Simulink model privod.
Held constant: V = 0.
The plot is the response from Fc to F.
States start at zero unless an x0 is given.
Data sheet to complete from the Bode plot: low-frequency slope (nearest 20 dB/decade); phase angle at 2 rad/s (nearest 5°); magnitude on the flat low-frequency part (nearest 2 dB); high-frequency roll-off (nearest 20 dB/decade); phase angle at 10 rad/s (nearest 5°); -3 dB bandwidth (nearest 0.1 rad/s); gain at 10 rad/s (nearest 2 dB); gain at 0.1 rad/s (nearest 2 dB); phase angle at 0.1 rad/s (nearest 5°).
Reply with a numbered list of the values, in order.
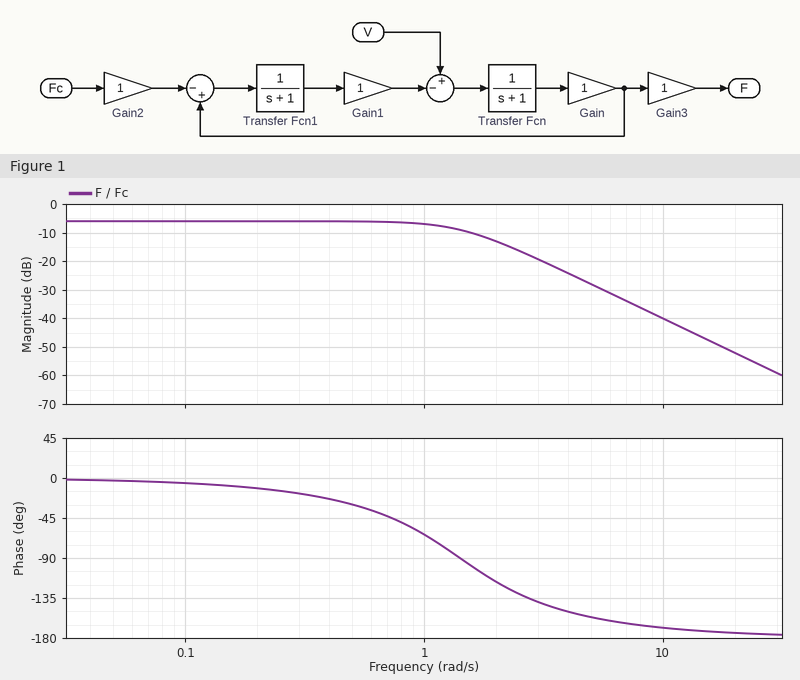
1. 0 dB/decade
2. -115°
3. -6 dB
4. -40 dB/decade
5. -170°
6. 1.4 rad/s
7. -40 dB
8. -6 dB
9. -5°
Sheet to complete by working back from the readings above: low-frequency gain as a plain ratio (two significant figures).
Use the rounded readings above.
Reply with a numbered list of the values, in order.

1. 0.50
